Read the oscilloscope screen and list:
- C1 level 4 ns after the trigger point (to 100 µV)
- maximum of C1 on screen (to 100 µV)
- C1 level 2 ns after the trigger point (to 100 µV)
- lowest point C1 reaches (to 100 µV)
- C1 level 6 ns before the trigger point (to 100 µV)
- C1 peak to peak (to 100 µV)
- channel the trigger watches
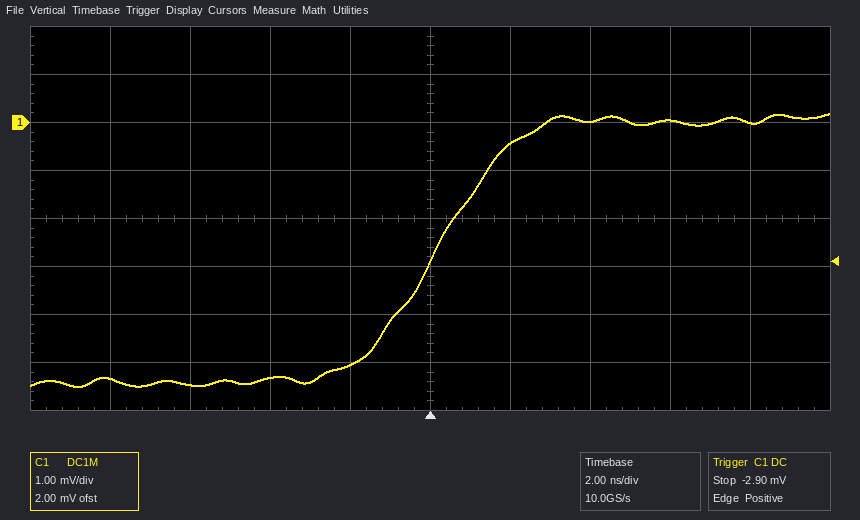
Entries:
0.0 mV
200 µV
-400 µV
-5.5 mV
-5.5 mV
5.7 mV
C1
